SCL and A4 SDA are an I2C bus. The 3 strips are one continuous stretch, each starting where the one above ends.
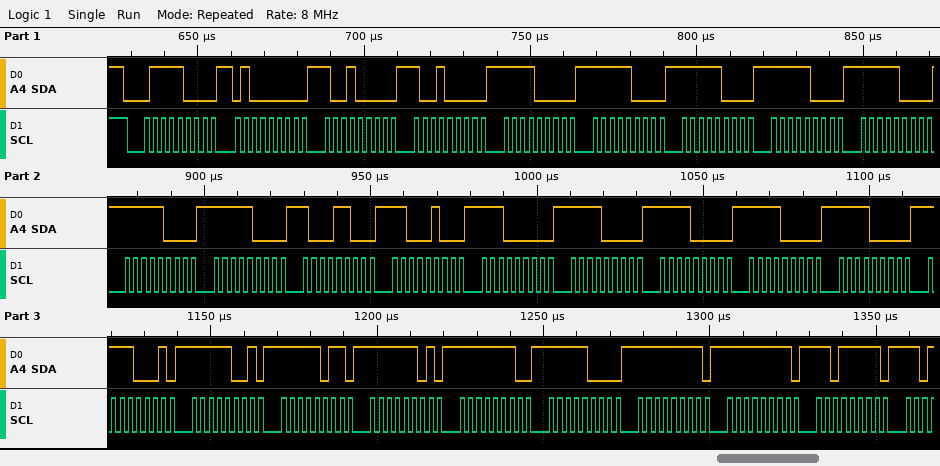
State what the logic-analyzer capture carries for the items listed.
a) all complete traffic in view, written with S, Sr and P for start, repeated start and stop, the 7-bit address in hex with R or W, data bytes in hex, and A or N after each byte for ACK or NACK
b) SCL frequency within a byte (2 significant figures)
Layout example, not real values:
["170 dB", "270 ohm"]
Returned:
["S 3CW A 40 A 90 A 90 A F0 A F8 A F8 A F8 A F8 A F8 A F8 A 8C A C4 A E0 A F0 A F0 A F0 A F0 A F1 A F9 A FB A FD A FE A F8 A FF A FF A DF A", "400 kHz"]
